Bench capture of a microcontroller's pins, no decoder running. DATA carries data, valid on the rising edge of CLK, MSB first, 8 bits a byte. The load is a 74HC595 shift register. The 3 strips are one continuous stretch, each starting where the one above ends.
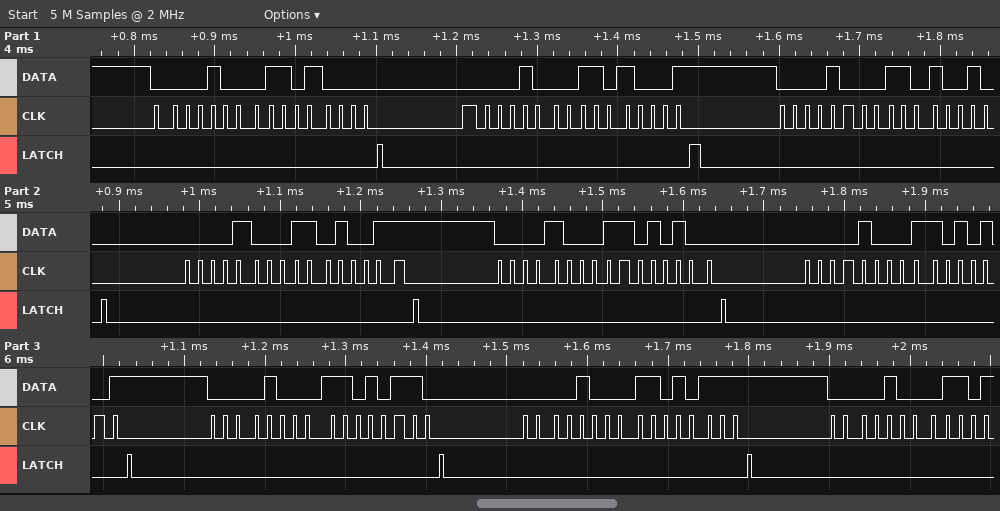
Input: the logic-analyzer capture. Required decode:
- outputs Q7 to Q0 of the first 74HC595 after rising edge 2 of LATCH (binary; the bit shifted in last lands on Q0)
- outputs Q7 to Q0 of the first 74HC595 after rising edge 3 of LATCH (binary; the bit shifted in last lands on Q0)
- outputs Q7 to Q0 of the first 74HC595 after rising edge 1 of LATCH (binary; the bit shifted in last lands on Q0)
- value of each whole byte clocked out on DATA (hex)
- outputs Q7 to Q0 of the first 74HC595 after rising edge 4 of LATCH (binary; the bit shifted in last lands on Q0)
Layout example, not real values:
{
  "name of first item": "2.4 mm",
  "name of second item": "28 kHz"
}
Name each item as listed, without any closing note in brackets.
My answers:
{
  "outputs Q7 to Q0 of the first 74HC595 after rising edge 2 of LATCH": "11010001",
  "outputs Q7 to Q0 of the first 74HC595 after rising edge 3 of LATCH": "11010010",
  "outputs Q7 to Q0 of the first 74HC595 after rising edge 1 of LATCH": "11010000",
  "value of each whole byte clocked out on DATA": "08 D0 08 D1 08 D2 08 D3 08 D4 08 D5 08 D6 08 D7 08",
  "outputs Q7 to Q0 of the first 74HC595 after rising edge 4 of LATCH": "11010011"
}
